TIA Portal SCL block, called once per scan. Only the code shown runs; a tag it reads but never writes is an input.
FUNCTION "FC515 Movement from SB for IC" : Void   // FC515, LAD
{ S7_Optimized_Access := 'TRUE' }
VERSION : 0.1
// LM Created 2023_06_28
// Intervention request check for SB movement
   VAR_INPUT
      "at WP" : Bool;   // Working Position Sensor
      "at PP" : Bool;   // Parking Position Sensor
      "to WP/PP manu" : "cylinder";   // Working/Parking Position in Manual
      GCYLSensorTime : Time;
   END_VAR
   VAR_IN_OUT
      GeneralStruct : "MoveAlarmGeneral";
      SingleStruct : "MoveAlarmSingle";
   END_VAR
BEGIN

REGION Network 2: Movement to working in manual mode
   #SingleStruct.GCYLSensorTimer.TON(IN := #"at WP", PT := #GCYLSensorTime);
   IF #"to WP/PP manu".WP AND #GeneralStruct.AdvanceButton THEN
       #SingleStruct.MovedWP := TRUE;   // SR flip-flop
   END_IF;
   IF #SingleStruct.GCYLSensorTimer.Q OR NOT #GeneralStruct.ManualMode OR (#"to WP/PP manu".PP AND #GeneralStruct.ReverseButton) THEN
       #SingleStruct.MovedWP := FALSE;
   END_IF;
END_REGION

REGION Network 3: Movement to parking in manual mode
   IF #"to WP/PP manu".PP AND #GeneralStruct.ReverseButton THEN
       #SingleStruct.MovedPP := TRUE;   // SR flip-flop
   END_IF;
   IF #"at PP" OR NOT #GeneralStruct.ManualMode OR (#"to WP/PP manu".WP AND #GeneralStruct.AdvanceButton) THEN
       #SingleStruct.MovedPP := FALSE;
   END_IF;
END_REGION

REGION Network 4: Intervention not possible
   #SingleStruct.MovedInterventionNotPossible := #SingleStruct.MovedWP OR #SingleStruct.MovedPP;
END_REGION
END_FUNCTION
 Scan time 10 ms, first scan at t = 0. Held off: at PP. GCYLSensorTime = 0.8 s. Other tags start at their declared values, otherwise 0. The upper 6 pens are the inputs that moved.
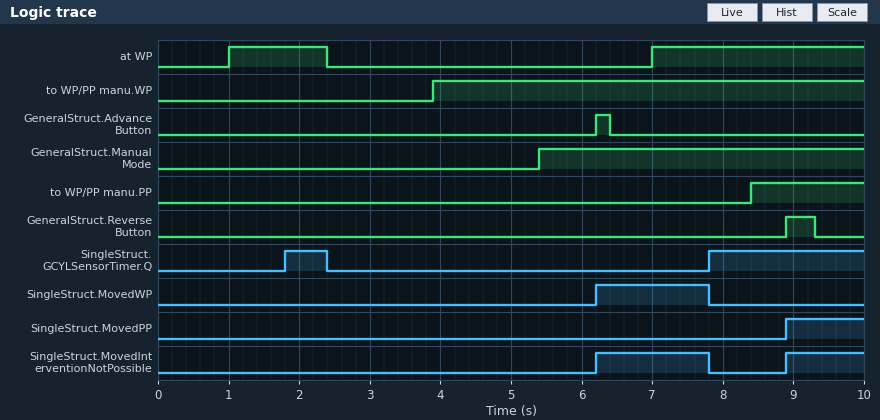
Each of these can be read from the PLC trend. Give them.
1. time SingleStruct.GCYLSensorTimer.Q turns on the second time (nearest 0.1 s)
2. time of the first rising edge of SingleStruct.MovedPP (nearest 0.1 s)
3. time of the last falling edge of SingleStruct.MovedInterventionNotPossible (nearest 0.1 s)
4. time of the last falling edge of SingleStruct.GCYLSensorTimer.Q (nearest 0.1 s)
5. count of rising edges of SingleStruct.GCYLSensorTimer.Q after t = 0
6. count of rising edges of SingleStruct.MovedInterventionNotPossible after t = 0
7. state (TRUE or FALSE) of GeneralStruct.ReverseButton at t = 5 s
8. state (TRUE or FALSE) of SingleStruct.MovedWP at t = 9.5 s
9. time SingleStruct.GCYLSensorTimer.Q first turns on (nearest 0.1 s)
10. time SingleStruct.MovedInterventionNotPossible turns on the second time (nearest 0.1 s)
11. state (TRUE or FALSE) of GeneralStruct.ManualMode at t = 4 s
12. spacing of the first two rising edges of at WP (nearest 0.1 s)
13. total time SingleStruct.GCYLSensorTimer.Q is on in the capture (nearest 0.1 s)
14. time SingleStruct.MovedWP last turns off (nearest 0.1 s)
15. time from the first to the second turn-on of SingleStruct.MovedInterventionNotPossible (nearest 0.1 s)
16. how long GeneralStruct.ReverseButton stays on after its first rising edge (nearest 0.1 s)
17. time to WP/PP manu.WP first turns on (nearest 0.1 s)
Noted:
7.8 s
8.9 s
7.8 s
2.4 s
2
2
FALSE
FALSE
1.8 s
8.9 s
FALSE
6.0 s
2.8 s
7.8 s
2.7 s
0.4 s
3.9 s
